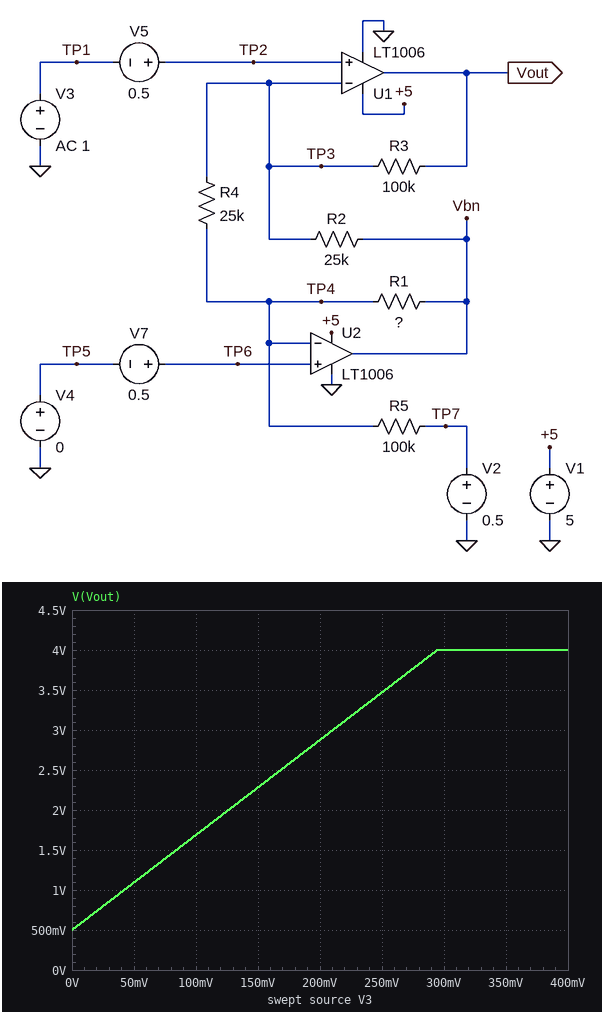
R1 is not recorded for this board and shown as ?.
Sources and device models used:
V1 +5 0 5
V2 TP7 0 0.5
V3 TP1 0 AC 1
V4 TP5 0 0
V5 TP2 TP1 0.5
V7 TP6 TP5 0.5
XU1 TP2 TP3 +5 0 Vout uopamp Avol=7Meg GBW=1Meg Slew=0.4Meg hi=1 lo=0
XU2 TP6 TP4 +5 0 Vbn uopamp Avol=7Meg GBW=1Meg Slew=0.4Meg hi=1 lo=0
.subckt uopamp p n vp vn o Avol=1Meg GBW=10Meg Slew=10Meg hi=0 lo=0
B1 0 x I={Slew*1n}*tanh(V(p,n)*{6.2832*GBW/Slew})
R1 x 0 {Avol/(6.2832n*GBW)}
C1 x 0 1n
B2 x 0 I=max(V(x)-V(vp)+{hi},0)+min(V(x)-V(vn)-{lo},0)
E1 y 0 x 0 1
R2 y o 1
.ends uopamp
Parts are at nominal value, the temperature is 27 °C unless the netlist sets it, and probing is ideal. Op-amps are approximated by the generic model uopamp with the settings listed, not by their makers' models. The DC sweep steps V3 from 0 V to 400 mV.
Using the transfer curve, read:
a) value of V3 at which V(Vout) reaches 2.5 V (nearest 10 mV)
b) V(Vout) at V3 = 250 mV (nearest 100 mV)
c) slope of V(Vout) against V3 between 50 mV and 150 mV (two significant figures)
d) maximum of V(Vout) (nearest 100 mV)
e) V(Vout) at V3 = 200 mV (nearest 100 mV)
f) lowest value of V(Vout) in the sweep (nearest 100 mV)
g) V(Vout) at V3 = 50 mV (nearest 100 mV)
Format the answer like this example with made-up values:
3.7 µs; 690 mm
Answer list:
170 mV; 3.5 V; 12 V/V; 4.0 V; 2.9 V; 500 mV; 1.1 V
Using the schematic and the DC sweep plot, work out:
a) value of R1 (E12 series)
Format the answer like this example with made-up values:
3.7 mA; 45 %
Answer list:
18 kΩ
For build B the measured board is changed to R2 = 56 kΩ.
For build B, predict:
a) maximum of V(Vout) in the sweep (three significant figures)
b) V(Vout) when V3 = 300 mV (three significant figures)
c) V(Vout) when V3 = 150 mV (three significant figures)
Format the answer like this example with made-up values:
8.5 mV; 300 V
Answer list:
3.73 V; 2.92 V; 1.71 V
